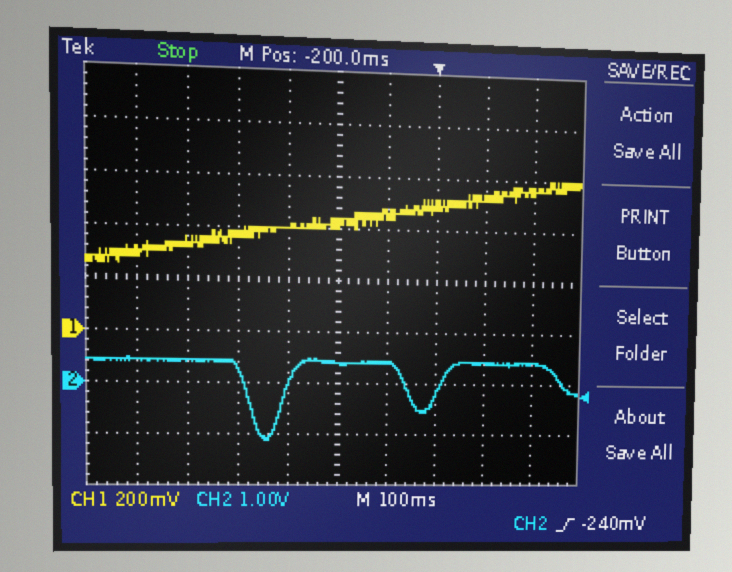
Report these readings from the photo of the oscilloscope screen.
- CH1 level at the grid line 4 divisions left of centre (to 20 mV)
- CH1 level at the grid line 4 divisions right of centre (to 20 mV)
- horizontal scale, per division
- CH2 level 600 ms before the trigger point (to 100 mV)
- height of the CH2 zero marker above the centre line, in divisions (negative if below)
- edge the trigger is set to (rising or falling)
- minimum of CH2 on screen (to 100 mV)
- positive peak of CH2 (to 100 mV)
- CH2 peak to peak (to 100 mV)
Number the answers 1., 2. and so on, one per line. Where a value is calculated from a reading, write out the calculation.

1. 300 mV
2. 560 mV
3. 100 ms
4. 400 mV
5. -2.0 div
6. rising
7. -1.1 V
8. 500 mV
9. 500 mV − (-1.1 V) = 1.6 V
